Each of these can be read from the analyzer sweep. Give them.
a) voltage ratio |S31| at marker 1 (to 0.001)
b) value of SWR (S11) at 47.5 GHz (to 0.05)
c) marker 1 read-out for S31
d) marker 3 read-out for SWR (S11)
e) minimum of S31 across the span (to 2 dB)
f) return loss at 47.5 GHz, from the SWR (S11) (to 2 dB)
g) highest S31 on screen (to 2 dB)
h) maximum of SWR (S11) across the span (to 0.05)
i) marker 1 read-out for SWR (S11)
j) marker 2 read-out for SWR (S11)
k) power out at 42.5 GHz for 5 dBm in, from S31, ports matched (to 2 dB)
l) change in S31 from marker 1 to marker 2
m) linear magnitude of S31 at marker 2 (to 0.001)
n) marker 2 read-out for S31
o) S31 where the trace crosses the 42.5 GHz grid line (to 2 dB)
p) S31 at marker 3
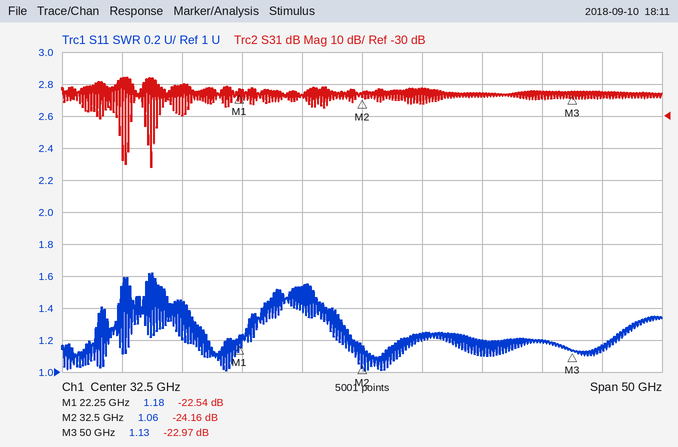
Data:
0.075
1.20
-22.54 dB
1.13
-46 dB
20 dB
-18 dB
1.60
1.18
1.06
-18 dBm
-1.62 dB
0.062
-24.16 dB
-24 dB
-22.97 dB
